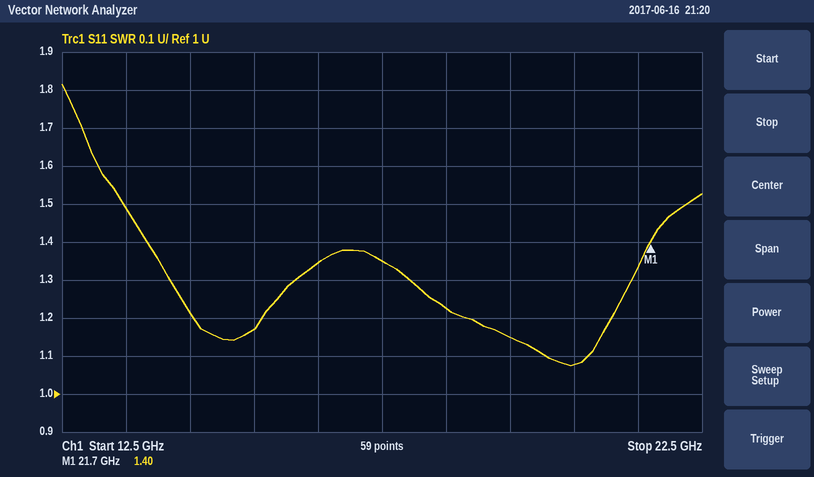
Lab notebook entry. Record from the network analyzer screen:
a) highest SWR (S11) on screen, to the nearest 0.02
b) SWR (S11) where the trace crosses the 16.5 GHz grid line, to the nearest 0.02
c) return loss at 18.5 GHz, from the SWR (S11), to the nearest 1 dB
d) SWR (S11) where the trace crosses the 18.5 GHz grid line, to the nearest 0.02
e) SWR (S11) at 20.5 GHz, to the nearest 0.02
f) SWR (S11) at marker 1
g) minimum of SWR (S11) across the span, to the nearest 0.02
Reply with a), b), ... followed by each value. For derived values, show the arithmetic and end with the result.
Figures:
a) 1.82
b) 1.34
c) −20 log10((1.22 − 1)/(1.22 + 1)) ≈ 20 dB
d) 1.22
e) 1.08
f) 1.40
g) 1.08
